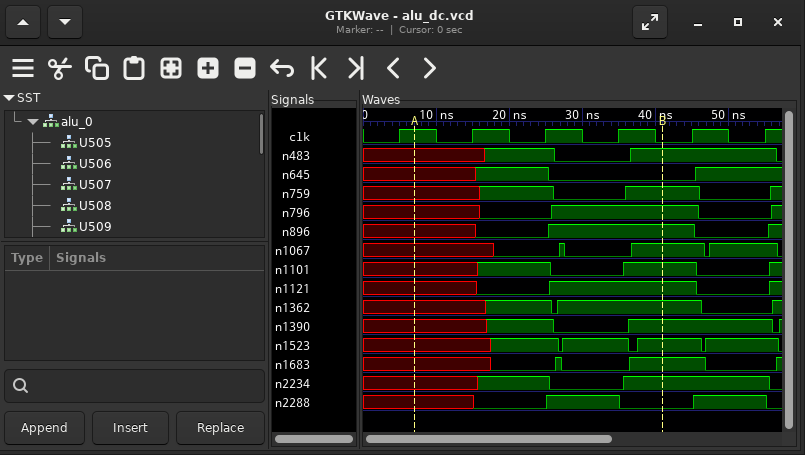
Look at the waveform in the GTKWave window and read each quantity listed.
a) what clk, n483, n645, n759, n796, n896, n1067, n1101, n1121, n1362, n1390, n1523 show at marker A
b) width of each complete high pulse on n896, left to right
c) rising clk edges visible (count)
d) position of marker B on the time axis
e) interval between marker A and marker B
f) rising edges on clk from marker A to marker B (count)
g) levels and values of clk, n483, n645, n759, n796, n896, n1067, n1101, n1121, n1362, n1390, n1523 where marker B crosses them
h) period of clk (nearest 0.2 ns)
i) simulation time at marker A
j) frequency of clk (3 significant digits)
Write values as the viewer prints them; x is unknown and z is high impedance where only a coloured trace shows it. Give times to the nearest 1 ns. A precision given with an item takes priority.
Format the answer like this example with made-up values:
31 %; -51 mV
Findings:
clk=1, n483=x, n645=x, n759=x, n796=x, n896=x, n1067=x, n1101=x, n1121=x, n1362=x, n1390=x, n1523=x; 20 ns; 6; 41 ns; 34 ns; 3; clk=0, n483=1, n645=0, n759=1, n796=1, n896=1, n1067=1, n1101=1, n1121=1, n1362=1, n1390=1, n1523=1; 10 ns; 7 ns; 100 MHz
